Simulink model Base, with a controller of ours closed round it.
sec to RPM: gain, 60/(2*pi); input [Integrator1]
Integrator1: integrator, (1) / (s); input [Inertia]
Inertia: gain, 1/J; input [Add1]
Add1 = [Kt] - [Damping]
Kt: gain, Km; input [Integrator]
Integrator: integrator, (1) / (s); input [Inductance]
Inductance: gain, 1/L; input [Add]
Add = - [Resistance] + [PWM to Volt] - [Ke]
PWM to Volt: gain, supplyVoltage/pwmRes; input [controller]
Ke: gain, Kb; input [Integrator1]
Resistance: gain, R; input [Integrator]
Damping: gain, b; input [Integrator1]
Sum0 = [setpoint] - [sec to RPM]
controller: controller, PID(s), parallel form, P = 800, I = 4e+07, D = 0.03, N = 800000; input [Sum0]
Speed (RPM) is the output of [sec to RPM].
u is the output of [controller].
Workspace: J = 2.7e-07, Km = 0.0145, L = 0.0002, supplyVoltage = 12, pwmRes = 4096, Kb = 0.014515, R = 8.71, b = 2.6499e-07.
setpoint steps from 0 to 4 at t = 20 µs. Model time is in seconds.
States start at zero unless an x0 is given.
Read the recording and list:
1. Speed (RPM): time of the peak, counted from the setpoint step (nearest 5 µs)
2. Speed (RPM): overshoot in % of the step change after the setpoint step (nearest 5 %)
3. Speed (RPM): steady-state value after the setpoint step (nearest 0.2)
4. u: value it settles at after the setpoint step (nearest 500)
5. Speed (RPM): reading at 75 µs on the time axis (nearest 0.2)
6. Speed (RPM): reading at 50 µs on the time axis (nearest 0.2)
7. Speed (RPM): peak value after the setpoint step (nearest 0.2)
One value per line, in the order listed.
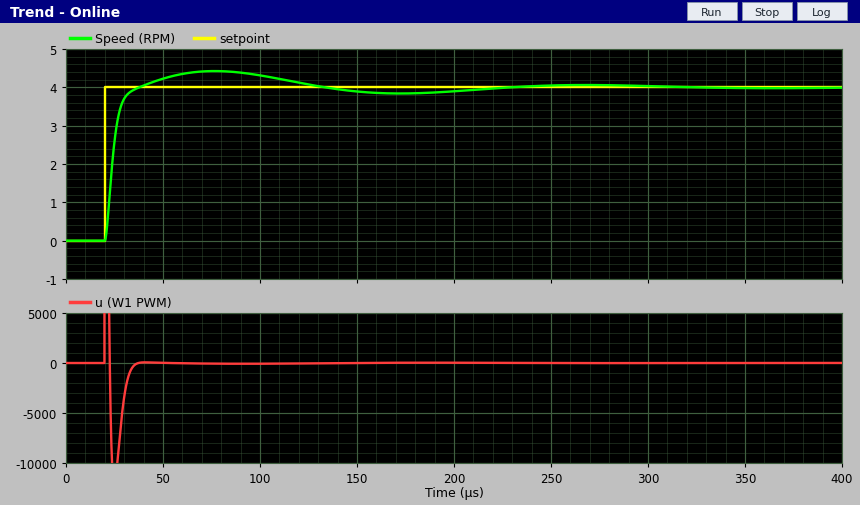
55 µs
10 %
4.0
0
4.4
4.2
4.4
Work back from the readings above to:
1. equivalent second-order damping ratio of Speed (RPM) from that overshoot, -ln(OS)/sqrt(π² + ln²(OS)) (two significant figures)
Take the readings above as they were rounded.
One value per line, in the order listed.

0.59
